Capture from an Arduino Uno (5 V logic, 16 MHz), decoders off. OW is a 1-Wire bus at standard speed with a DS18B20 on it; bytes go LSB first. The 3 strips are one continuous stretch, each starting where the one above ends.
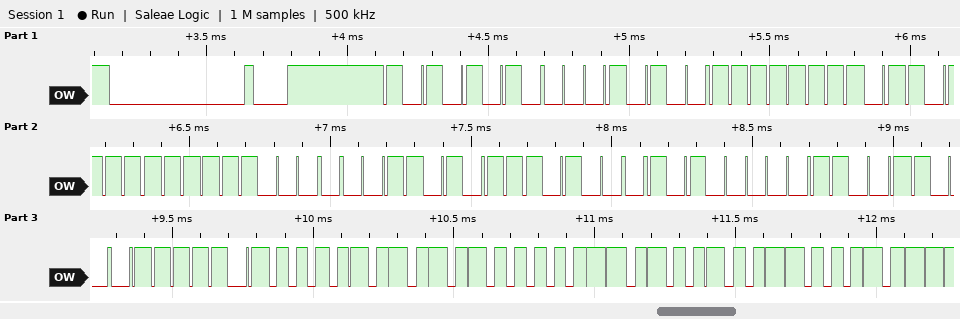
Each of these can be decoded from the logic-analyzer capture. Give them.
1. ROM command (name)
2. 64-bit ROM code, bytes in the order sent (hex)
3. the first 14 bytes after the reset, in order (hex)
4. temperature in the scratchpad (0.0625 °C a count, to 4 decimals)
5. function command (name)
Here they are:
Match ROM
28 FF F6 1F 58 17 05 33
55 28 FF F6 1F 58 17 05 33 BE 50 05 4B 46
85.0000 °C
Read Scratchpad
